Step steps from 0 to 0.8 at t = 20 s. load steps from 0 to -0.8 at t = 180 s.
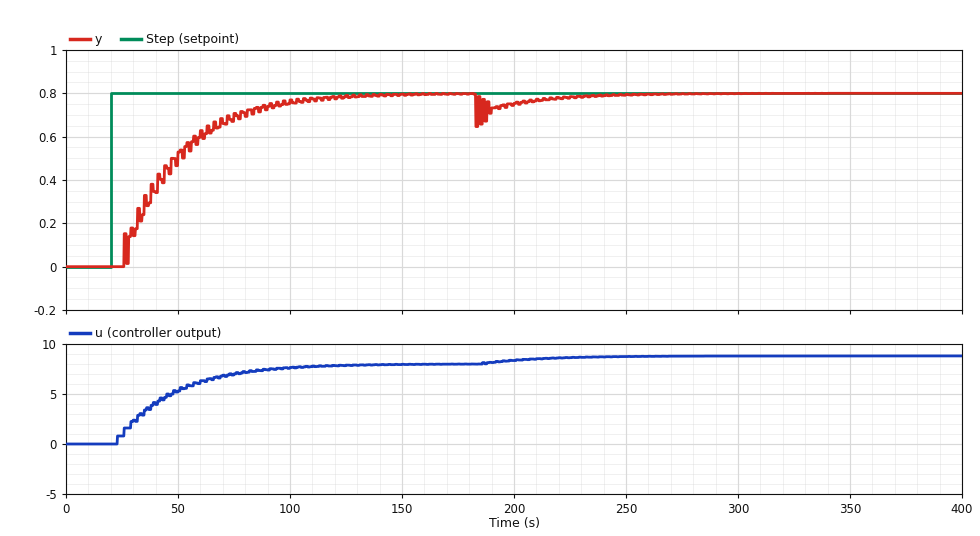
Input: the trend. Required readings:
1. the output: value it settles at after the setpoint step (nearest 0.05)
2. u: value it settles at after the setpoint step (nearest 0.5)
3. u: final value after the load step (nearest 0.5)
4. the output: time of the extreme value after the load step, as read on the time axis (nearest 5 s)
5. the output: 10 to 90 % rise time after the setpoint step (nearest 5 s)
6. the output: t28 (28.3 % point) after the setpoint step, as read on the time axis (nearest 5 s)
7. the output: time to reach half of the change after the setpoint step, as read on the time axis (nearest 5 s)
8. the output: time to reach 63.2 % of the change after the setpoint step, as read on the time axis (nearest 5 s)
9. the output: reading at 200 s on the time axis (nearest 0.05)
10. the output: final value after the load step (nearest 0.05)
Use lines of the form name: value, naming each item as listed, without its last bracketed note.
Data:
the output: value it settles at after the setpoint step: 0.80
u: value it settles at after the setpoint step: 8.0
u: final value after the load step: 9.0
the output: time of the extreme value after the load step, as read on the time axis: 185 s
the output: 10 to 90 % rise time after the setpoint step: 55 s
the output: t28 (28.3 % point) after the setpoint step, as read on the time axis: 30 s
the output: time to reach half of the change after the setpoint step, as read on the time axis: 40 s
the output: time to reach 63.2 % of the change after the setpoint step, as read on the time axis: 50 s
the output: reading at 200 s on the time axis: 0.75
the output: final value after the load step: 0.80
